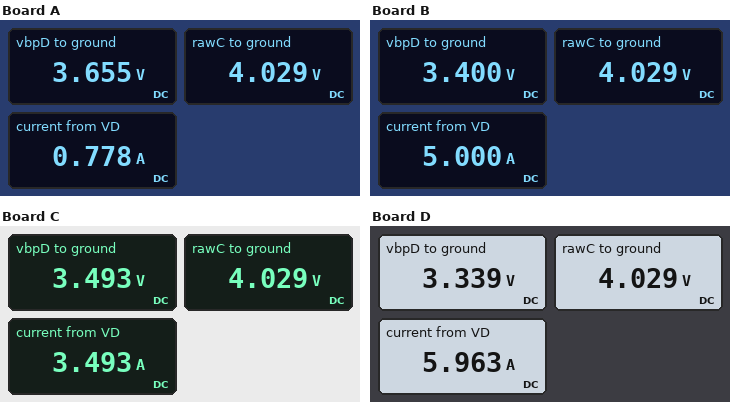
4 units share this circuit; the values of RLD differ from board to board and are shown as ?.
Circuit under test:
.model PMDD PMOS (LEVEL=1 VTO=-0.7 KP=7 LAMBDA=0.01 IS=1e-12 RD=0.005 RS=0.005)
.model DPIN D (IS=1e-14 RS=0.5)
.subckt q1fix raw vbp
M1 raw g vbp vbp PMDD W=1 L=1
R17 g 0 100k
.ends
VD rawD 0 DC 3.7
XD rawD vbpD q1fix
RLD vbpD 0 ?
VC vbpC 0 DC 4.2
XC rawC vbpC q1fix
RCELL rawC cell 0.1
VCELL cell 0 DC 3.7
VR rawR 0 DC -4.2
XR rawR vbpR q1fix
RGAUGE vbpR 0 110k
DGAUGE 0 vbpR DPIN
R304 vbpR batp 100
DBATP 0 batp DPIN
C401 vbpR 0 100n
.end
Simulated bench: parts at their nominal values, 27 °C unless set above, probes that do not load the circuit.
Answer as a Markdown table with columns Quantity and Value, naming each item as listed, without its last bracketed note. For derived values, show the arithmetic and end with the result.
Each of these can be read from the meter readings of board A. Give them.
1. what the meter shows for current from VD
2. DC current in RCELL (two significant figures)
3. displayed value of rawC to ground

| Quantity | Value |
|---|---|
| what the meter shows for current from VD | 0.778 A |
| DC current in RCELL | (4.029 V - 3.7 V) / 100 mΩ = 3.3 A |
| displayed value of rawC to ground | 4.029 V |
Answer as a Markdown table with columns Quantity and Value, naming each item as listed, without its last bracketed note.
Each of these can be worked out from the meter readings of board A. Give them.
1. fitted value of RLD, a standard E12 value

| Quantity | Value |
|---|---|
| fitted value of RLD, a standard E12 value | 4.7 Ω |
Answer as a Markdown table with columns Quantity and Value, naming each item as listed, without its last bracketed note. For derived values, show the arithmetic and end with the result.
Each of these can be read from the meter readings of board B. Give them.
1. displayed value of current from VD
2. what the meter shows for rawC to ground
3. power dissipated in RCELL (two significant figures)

| Quantity | Value |
|---|---|
| displayed value of current from VD | 5.000 A |
| what the meter shows for rawC to ground | 4.029 V |
| power dissipated in RCELL | (4.029 V - 3.7 V)^2 / 100 mΩ = 1.1 W |
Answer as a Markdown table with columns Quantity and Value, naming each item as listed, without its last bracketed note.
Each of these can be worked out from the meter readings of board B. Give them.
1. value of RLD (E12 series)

| Quantity | Value |
|---|---|
| value of RLD | 0.68 Ω |
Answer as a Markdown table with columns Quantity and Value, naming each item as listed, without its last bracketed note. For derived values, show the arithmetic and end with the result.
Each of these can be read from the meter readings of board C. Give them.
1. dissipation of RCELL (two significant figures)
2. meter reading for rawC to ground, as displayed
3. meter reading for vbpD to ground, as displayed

| Quantity | Value |
|---|---|
| dissipation of RCELL | (4.029 V - 3.7 V)^2 / 100 mΩ = 1.1 W |
| meter reading for rawC to ground, as displayed | 4.029 V |
| meter reading for vbpD to ground, as displayed | 3.493 V |
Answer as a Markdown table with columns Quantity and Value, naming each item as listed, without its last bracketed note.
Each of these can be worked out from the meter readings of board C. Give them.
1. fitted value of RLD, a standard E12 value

| Quantity | Value |
|---|---|
| fitted value of RLD, a standard E12 value | 1 Ω |
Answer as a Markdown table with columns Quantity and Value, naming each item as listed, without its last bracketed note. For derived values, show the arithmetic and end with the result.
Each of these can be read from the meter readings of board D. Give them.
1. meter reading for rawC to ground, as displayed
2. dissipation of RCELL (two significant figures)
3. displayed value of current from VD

| Quantity | Value |
|---|---|
| meter reading for rawC to ground, as displayed | 4.029 V |
| dissipation of RCELL | (4.029 V - 3.7 V)^2 / 100 mΩ = 1.1 W |
| displayed value of current from VD | 5.963 A |
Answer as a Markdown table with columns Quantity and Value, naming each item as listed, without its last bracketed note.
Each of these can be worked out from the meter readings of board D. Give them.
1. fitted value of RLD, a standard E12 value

| Quantity | Value |
|---|---|
| fitted value of RLD, a standard E12 value | 0.56 Ω |
